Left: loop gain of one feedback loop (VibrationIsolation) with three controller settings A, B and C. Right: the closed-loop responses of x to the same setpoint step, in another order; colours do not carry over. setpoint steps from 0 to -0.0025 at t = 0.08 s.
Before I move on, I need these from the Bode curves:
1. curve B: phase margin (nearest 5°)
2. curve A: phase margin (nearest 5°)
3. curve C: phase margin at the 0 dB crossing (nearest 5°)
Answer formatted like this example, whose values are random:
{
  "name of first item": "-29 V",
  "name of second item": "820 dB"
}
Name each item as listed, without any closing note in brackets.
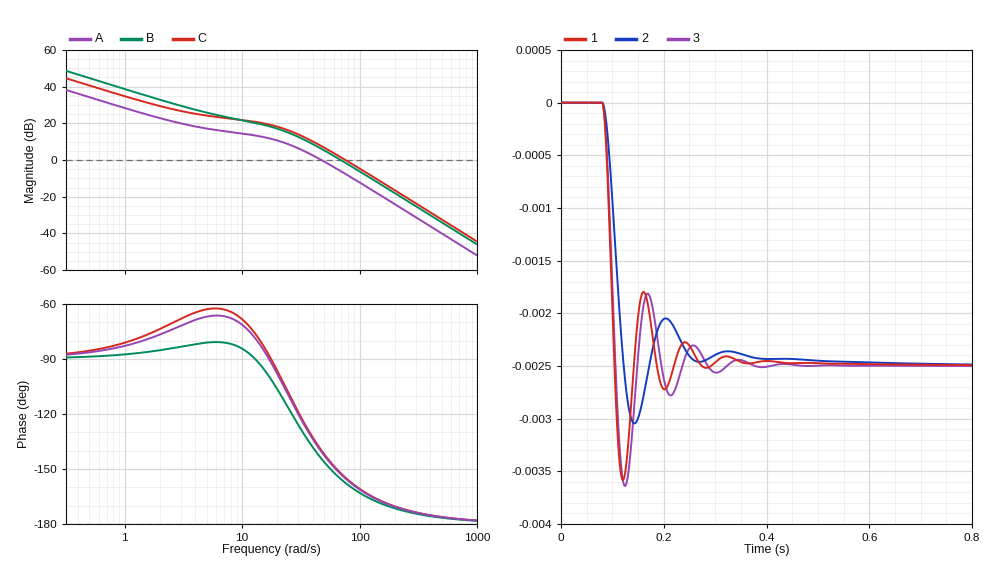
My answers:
{
  "curve B: phase margin": "25°",
  "curve A: phase margin": "40°",
  "curve C: phase margin at the 0 dB crossing": "25°"
}
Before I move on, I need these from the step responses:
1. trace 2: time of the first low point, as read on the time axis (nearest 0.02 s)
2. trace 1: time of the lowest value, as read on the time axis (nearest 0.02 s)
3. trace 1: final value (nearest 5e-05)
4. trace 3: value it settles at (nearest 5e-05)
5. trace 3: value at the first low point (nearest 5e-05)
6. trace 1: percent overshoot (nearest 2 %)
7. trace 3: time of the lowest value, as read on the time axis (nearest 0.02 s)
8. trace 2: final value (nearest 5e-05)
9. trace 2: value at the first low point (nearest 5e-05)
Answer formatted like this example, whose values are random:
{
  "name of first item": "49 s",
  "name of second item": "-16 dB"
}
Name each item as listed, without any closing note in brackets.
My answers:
{
  "trace 2: time of the first low point, as read on the time axis": "0.14 s",
  "trace 1: time of the lowest value, as read on the time axis": "0.12 s",
  "trace 1: final value": "-0.00250",
  "trace 3: value it settles at": "-0.00250",
  "trace 3: value at the first low point": "-0.00365",
  "trace 1: percent overshoot": "44 %",
  "trace 3: time of the lowest value, as read on the time axis": "0.12 s",
  "trace 2: final value": "-0.00250",
  "trace 2: value at the first low point": "-0.00305"
}
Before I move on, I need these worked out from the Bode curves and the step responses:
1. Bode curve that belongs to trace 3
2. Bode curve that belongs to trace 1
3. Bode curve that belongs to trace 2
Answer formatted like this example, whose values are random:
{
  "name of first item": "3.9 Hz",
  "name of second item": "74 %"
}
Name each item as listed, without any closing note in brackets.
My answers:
{
  "Bode curve that belongs to trace 3": "B",
  "Bode curve that belongs to trace 1": "C",
  "Bode curve that belongs to trace 2": "A"
}
